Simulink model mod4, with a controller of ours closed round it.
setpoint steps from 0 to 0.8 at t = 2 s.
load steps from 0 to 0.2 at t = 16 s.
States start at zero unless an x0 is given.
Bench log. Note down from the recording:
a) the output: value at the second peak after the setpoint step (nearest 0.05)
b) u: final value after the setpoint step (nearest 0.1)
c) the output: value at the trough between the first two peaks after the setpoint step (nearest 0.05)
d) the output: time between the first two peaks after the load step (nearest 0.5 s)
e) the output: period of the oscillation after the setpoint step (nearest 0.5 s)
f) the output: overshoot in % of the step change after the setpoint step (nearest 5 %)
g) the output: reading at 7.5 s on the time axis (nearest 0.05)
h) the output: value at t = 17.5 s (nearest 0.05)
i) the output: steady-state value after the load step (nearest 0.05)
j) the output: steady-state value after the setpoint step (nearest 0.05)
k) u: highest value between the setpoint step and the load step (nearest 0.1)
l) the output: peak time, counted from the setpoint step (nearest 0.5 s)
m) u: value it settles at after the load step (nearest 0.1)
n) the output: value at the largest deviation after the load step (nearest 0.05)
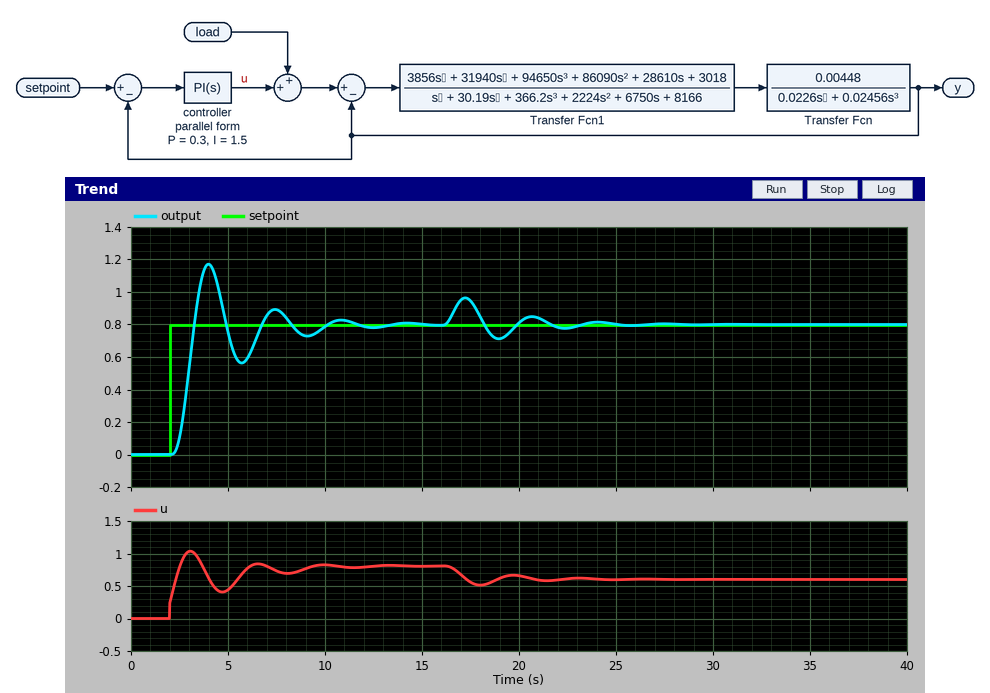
0.90
0.8
0.55
3.5 s
3.5 s
45 %
0.90
0.95
0.80
0.80
1.0
2.0 s
0.6
0.95
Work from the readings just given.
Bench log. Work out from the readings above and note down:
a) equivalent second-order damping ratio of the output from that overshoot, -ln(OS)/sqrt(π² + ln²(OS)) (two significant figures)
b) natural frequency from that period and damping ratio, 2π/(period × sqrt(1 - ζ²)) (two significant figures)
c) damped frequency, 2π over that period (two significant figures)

0.25
1.9 rad/s
1.8 rad/s
